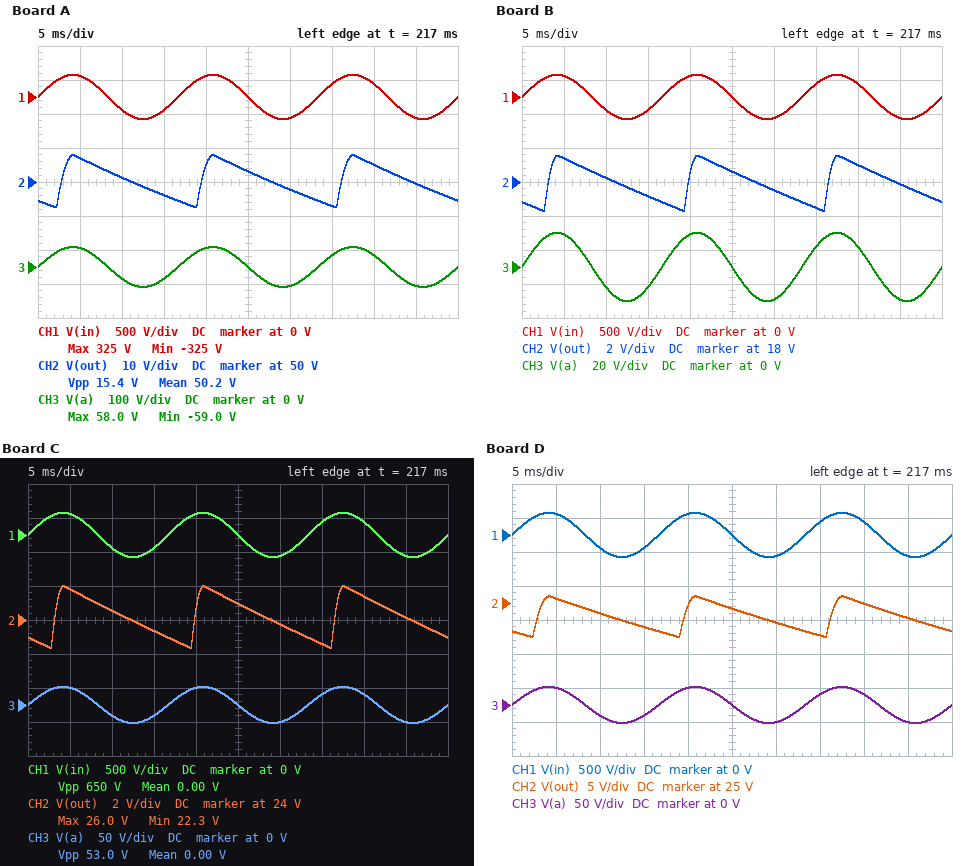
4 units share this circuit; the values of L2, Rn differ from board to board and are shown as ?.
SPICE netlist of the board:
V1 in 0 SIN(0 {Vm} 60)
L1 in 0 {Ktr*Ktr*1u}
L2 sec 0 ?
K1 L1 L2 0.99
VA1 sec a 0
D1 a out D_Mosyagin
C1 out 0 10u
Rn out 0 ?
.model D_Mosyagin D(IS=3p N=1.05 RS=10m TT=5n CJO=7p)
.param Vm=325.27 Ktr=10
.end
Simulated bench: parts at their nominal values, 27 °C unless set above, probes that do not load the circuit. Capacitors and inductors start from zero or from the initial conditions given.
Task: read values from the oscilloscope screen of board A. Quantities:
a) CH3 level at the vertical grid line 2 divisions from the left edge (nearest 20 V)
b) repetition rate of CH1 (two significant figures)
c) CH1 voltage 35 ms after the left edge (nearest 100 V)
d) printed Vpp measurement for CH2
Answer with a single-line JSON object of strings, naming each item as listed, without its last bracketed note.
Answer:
{"CH3 level at the vertical grid line 2 divisions from the left edge": "-40 V", "repetition rate of CH1": "60 Hz", "CH1 voltage 35 ms after the left edge": "200 V", "printed Vpp measurement for CH2": "15.4 V"}
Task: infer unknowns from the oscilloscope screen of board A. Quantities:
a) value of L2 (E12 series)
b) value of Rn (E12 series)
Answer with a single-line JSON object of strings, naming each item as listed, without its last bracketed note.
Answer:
{"value of L2": "3.3 µH", "value of Rn": "4.7 kΩ"}
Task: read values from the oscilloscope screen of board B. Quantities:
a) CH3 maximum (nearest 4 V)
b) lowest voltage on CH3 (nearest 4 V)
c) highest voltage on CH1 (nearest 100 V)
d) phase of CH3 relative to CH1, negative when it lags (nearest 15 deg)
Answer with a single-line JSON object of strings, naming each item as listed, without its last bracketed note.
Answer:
{"CH3 maximum": "20 V", "lowest voltage on CH3": "-20 V", "highest voltage on CH1": "300 V", "phase of CH3 relative to CH1, negative when it lags": "0 deg"}
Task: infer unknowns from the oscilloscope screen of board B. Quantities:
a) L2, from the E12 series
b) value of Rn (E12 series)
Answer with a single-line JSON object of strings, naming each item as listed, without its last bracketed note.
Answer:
{"L2, from the E12 series": "390 nH", "value of Rn": "8.2 kΩ"}
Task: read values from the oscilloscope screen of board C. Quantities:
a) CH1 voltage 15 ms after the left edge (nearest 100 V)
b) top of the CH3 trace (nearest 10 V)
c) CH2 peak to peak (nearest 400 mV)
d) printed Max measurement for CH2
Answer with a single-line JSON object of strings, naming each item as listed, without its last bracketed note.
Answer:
{"CH1 voltage 15 ms after the left edge": "-200 V", "top of the CH3 trace": "30 V", "CH2 peak to peak": "3.6 V", "printed Max measurement for CH2": "26.0 V"}
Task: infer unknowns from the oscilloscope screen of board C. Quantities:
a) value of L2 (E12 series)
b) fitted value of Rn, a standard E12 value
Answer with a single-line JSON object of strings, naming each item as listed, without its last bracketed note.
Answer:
{"value of L2": "680 nH", "fitted value of Rn, a standard E12 value": "10 kΩ"}
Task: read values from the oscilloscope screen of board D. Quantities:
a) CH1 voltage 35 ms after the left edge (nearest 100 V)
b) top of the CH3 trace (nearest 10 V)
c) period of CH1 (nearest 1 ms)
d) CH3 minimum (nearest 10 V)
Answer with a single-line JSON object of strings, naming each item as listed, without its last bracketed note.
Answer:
{"CH1 voltage 35 ms after the left edge": "200 V", "top of the CH3 trace": "30 V", "period of CH1": "17 ms", "CH3 minimum": "-30 V"}
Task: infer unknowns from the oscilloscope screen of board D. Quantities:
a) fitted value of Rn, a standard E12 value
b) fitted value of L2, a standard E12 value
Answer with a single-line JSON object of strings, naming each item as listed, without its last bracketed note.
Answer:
{"fitted value of Rn, a standard E12 value": "5.6 kΩ", "fitted value of L2, a standard E12 value": "680 nH"}
